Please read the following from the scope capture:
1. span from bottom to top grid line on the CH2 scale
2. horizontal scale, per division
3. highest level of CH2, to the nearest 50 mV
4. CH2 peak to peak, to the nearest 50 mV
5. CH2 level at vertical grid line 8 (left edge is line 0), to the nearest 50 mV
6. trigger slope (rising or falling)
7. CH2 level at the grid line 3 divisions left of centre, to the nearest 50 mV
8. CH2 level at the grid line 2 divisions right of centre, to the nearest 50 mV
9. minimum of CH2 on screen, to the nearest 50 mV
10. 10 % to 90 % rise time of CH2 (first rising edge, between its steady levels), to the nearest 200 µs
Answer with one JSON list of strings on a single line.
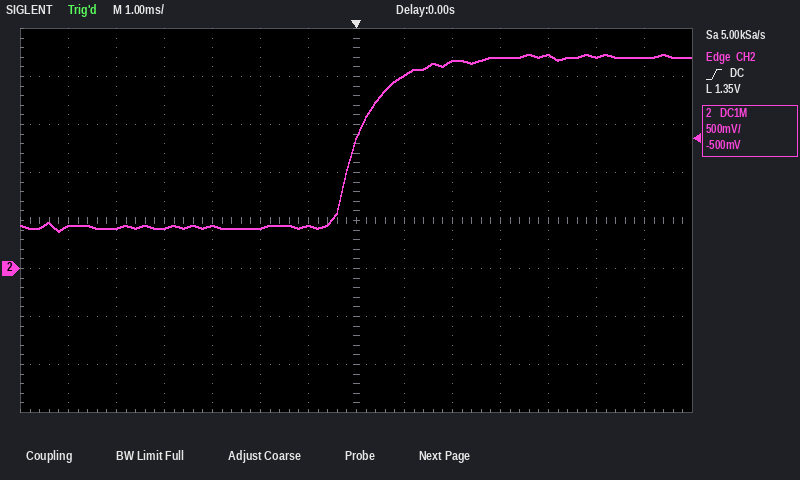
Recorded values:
["4 V", "1 ms", "2.25 V", "1.85 V", "2.00 V", "rising", "450 mV", "2.15 V", "400 mV", "1.4 ms"]
